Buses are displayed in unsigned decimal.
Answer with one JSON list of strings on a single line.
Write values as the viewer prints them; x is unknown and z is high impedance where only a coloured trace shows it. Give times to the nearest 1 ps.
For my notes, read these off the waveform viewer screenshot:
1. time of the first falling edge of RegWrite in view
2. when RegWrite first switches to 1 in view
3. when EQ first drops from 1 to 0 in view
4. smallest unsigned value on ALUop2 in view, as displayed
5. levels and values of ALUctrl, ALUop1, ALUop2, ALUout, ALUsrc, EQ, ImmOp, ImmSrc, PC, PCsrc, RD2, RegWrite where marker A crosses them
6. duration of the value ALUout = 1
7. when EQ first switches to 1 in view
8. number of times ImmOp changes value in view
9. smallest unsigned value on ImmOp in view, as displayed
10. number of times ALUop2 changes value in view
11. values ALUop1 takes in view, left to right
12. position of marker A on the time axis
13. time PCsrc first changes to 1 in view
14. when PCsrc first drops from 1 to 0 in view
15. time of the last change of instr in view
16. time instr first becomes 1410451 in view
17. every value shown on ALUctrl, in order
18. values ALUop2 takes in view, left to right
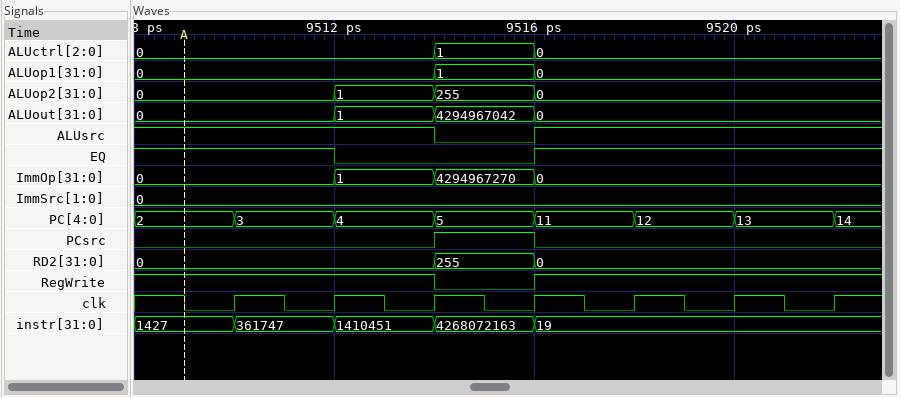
["9514 ps", "9516 ps", "9512 ps", "0", "ALUctrl=0, ALUop1=0, ALUop2=0, ALUout=0, ALUsrc=1, EQ=1, ImmOp=0, ImmSrc=0, PC=2, PCsrc=0, RD2=0, RegWrite=1", "2 ps", "9516 ps", "3", "0", "3", "0, 1, 0", "9509 ps", "9514 ps", "9516 ps", "9516 ps", "9512 ps", "0, 1, 0", "0, 1, 255, 0"]
